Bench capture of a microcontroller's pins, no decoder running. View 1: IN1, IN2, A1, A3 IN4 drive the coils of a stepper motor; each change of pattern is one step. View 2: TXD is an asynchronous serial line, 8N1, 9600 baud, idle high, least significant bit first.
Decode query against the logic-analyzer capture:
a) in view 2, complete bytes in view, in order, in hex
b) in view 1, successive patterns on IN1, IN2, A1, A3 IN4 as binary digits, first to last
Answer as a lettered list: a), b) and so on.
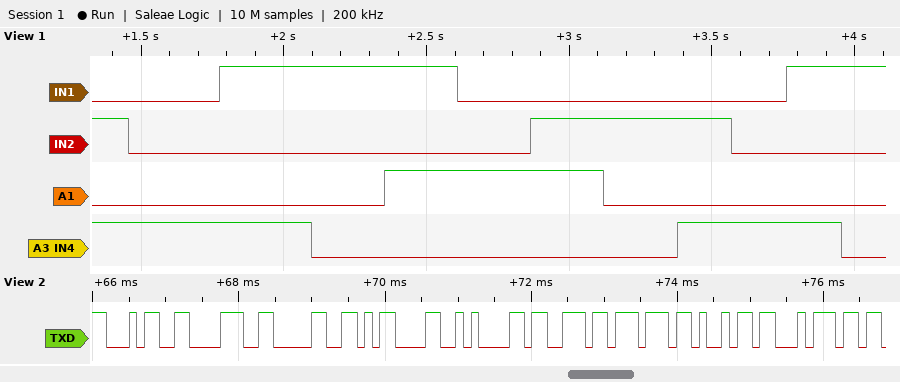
a) 34 38 30 0D 0A 73 77 69 74
b) 0101 0001 1001 1000 1010 0010 0110 0100 0101 0001 1001 1000
